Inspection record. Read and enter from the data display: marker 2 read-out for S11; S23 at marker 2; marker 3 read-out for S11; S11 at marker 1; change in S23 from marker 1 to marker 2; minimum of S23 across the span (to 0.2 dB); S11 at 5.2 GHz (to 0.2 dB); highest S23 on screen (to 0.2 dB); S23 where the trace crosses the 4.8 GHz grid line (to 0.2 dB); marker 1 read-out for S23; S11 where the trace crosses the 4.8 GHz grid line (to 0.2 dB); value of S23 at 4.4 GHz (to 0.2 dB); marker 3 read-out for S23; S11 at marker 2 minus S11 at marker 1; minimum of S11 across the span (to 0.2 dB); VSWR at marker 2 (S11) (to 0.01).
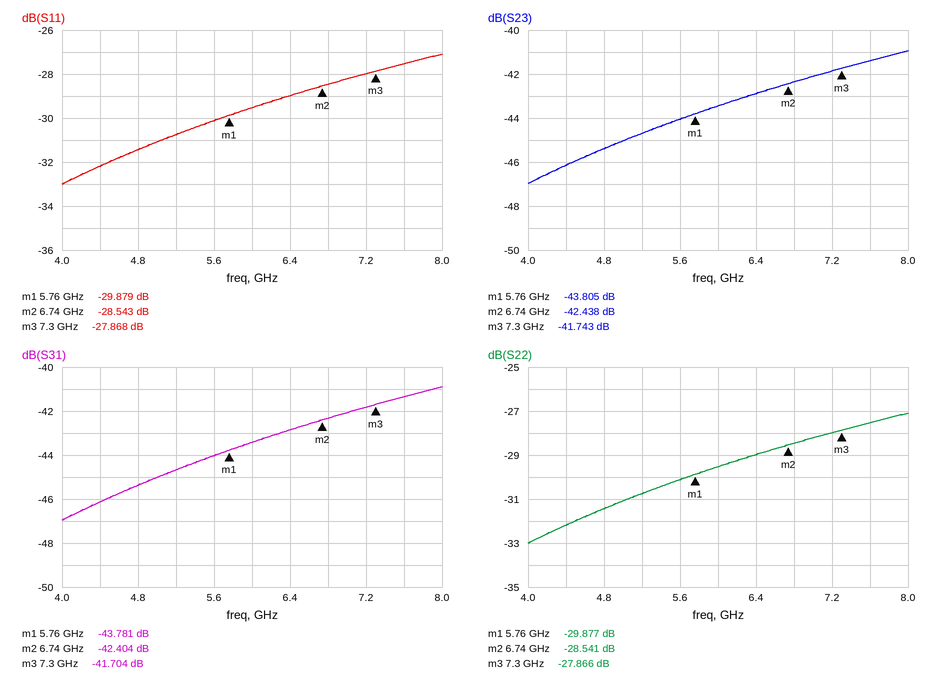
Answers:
-28.543 dB
-42.438 dB
-27.868 dB
-29.879 dB
1.367 dB
-47.0 dB
-30.8 dB
-41.0 dB
-45.4 dB
-43.805 dB
-31.4 dB
-46.2 dB
-41.743 dB
1.336 dB
-33.0 dB
1.08
